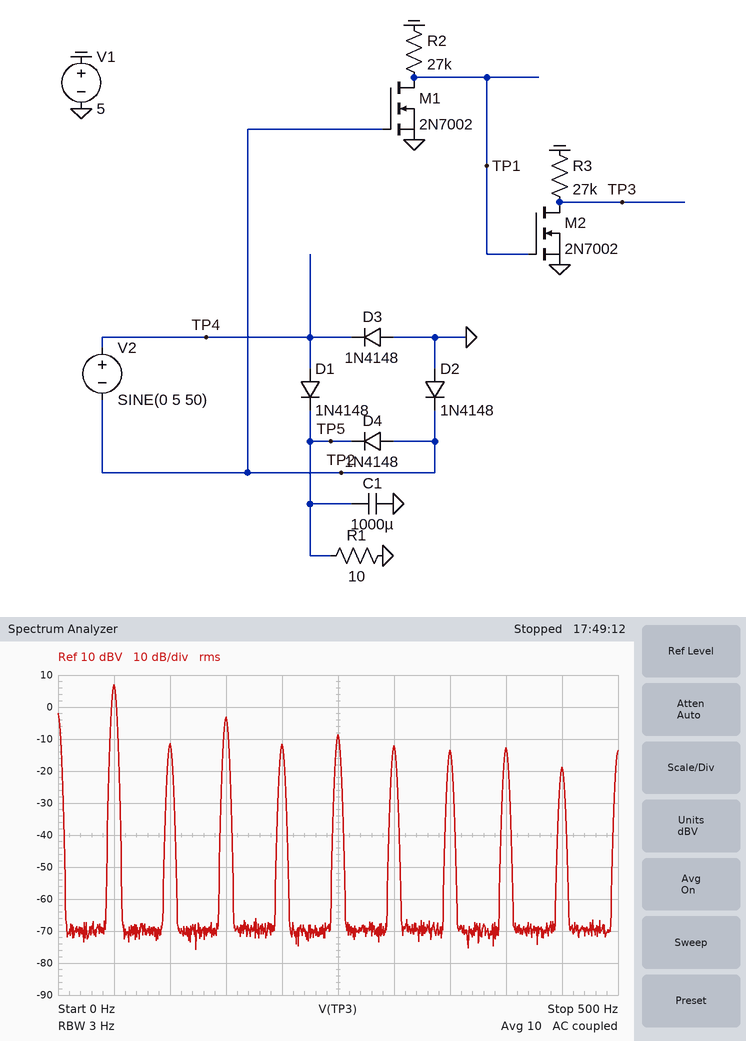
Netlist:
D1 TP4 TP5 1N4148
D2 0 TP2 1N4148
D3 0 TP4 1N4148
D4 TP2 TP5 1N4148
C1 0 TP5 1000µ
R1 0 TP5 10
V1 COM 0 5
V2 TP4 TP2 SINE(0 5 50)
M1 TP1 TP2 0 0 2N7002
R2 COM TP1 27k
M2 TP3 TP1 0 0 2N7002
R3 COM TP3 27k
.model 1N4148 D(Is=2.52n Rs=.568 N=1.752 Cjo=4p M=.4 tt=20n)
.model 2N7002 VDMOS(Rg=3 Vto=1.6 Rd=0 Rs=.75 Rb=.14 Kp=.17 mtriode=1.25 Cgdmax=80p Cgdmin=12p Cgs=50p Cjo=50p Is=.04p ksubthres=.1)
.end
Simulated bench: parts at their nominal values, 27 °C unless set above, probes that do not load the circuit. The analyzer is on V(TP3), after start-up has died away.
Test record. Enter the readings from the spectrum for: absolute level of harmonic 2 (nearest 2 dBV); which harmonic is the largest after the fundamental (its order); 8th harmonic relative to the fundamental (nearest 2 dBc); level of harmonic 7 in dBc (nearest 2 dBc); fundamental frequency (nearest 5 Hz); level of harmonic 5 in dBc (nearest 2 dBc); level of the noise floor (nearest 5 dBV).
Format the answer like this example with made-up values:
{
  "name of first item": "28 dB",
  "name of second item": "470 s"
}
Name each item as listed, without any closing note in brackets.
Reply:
{
  "absolute level of harmonic 2": "-12 dBV",
  "which harmonic is the largest after the fundamental": "3",
  "8th harmonic relative to the fundamental": "-20 dBc",
  "level of harmonic 7 in dBc": "-20 dBc",
  "fundamental frequency": "50 Hz",
  "level of harmonic 5 in dBc": "-16 dBc",
  "level of the noise floor": "-70 dBV"
}
